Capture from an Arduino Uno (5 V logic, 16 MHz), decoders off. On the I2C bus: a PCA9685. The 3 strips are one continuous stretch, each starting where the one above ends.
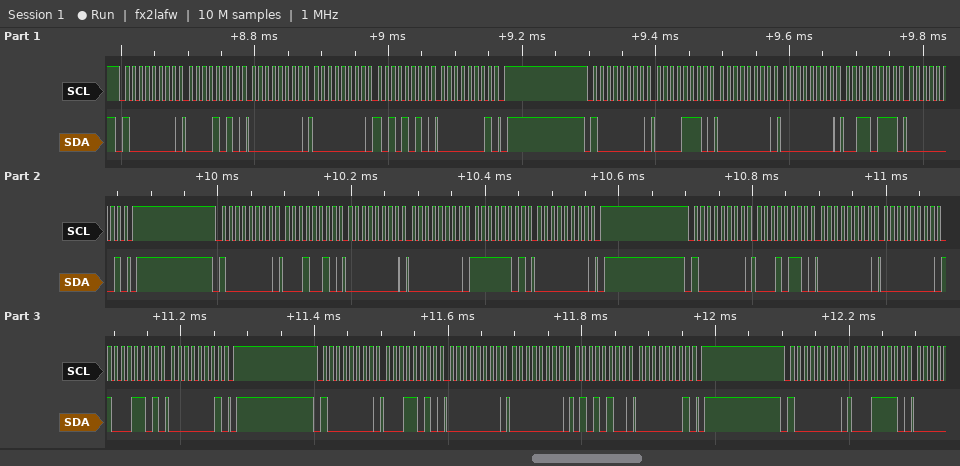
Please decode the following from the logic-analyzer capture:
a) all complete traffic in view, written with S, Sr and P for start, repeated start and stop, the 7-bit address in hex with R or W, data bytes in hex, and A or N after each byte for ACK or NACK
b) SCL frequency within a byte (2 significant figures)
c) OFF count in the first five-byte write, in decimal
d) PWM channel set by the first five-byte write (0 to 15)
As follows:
S 40W A 0A A 00 A 00 A AA A 01 A P S 40W A 0E A 00 A 00 A 37 A 01 A P S 40W A 12 A 00 A 00 A FD A 00 A P S 40W A 16 A 00 A 00 A 8D A 01 A P S 40W A 1A A 00 A 00 A 54 A 01 A P S 40W A 1E A
100 kHz
426
1
